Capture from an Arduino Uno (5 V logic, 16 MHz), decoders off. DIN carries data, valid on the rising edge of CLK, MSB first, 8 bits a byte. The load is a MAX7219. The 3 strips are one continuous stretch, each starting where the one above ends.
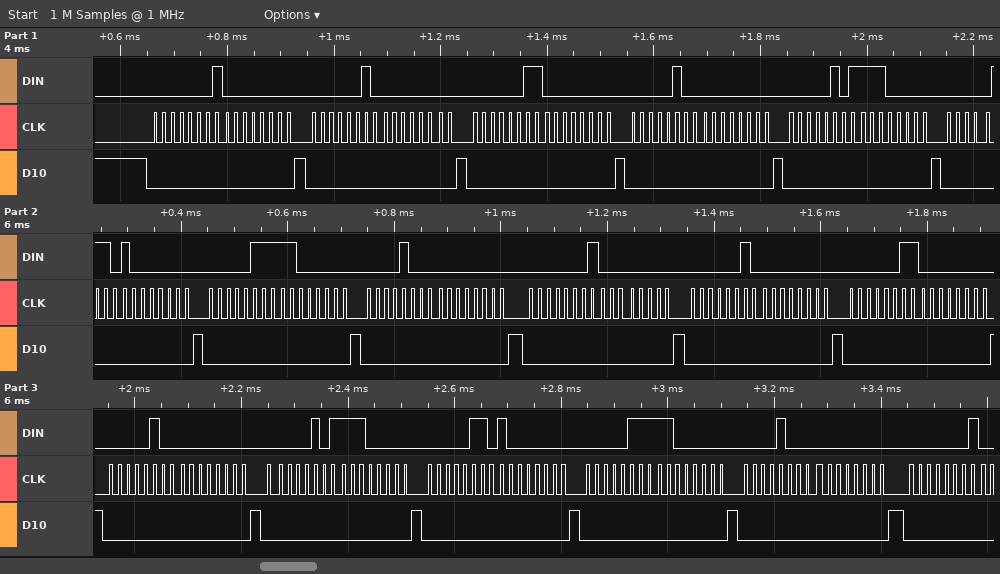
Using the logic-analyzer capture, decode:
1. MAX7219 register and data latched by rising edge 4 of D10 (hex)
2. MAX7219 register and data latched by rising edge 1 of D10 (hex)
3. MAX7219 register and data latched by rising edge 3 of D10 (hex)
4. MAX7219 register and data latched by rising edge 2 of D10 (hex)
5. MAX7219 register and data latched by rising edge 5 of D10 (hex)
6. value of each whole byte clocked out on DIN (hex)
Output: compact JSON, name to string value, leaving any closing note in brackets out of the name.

{"MAX7219 register and data latched by rising edge 4 of D10": "register 0x4, data 0x00", "MAX7219 register and data latched by rising edge 1 of D10": "register 0x1, data 0x00", "MAX7219 register and data latched by rising edge 3 of D10": "register 0x3, data 0x00", "MAX7219 register and data latched by rising edge 2 of D10": "register 0x2, data 0x00", "MAX7219 register and data latched by rising edge 5 of D10": "register 0x5, data 0xE0", "value of each whole byte clocked out on DIN": "01 00 02 00 03 00 04 00 05 E0 06 80 07 C0 08 00 01 00 02 00 03 00 04 00 05 E0 06 80 07 C0 08 00 01"}
